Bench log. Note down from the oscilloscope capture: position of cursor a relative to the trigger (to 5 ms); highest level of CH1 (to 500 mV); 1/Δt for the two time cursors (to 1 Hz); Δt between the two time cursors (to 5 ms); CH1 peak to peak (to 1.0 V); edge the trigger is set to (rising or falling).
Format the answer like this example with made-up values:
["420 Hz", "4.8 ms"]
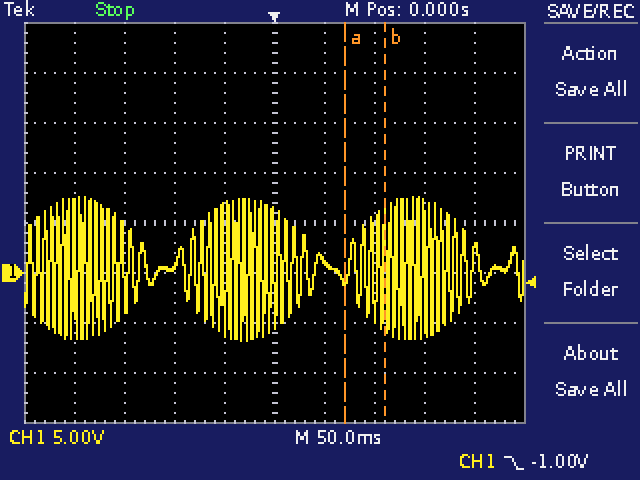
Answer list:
["+70 ms", "7.5 V", "25 Hz", "40 ms", "14.0 V", "falling"]
